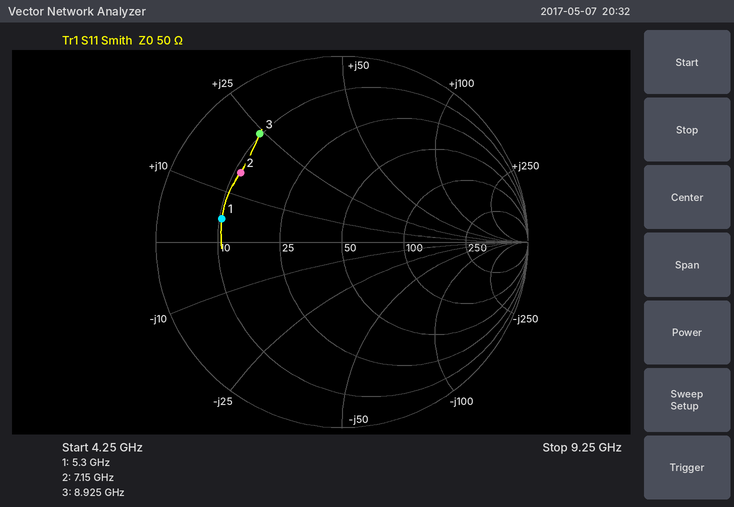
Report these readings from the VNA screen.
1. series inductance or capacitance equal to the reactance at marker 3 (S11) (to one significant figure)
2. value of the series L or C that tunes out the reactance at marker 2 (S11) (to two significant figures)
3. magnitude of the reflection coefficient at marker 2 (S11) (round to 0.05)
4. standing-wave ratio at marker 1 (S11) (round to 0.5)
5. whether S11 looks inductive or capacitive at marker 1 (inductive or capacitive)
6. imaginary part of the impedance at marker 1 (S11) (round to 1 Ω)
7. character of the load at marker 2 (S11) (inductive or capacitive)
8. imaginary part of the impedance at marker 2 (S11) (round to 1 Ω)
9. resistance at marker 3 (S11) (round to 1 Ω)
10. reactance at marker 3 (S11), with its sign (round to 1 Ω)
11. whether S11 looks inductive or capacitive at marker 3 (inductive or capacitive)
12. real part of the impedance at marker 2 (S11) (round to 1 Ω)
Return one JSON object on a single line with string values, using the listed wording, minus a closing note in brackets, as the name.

{"series inductance or capacitance equal to the reactance at marker 3 (S11)": "400 pH", "value of the series L or C that tunes out the reactance at marker 2 (S11)": "1.5 pF", "magnitude of the reflection coefficient at marker 2 (S11)": "0.65", "standing-wave ratio at marker 1 (S11)": "5.0", "whether S11 looks inductive or capacitive at marker 1": "inductive", "imaginary part of the impedance at marker 1 (S11)": "+5 Ω", "character of the load at marker 2 (S11)": "inductive", "imaginary part of the impedance at marker 2 (S11)": "+15 Ω", "resistance at marker 3 (S11)": "10 Ω", "reactance at marker 3 (S11), with its sign": "+24 Ω", "whether S11 looks inductive or capacitive at marker 3": "inductive", "real part of the impedance at marker 2 (S11)": "11 Ω"}
